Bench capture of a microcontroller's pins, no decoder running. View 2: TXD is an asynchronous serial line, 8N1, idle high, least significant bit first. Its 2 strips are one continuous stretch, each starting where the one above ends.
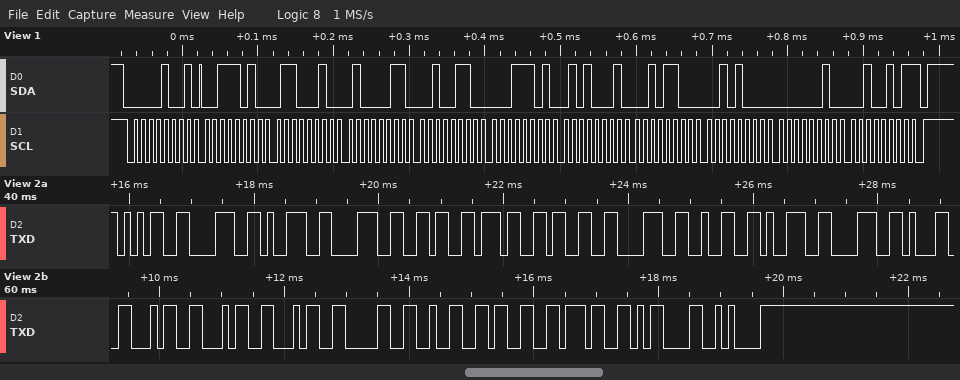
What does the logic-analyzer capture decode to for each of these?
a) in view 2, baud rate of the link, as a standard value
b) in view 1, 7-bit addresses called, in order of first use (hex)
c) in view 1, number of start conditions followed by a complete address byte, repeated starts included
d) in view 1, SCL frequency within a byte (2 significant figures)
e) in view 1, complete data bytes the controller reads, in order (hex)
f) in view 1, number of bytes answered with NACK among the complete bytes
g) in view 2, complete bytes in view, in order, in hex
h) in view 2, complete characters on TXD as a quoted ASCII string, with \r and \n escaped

9600 baud
0x04
1
100 kHz
3A 62 43 26 1D 51 2C 28 02 25
1
35 38 39 38 36 37 33 38 32 39 38 31 34 34 34 30 32 33 37 0D 0A
"5898673829814440237\r\n"
